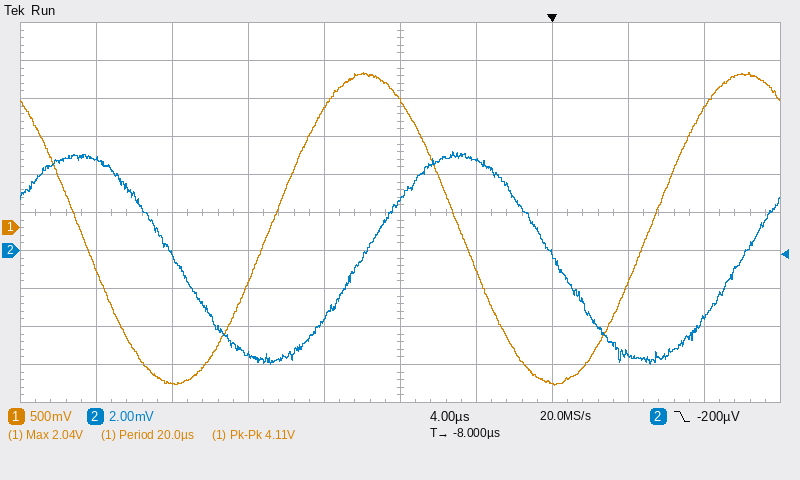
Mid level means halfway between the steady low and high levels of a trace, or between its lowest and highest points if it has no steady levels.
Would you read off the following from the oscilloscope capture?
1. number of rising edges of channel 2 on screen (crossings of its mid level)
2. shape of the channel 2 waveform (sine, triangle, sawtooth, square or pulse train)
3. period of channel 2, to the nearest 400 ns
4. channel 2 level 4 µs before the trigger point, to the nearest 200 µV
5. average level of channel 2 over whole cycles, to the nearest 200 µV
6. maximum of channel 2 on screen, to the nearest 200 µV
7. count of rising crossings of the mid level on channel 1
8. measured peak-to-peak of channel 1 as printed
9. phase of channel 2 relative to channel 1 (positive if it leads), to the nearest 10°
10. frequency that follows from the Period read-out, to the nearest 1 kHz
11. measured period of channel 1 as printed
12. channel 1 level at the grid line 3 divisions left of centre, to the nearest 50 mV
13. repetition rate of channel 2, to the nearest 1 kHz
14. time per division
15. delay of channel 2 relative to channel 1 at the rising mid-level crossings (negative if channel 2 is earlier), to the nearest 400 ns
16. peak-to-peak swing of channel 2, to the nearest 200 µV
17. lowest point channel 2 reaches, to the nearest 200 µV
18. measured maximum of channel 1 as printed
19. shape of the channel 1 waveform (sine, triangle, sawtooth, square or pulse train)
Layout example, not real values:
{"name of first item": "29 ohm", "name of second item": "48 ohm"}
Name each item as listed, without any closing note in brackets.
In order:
{"number of rising edges of channel 2 on screen": "2", "shape of the channel 2 waveform": "sine", "period of channel 2, to the nearest 400 ns": "20.0 µs", "channel 2 level 4 µs before the trigger point, to the nearest 200 µV": "4.8 mV", "average level of channel 2 over whole cycles, to the nearest 200 µV": "-400 µV", "maximum of channel 2 on screen, to the nearest 200 µV": "5.2 mV", "count of rising crossings of the mid level on channel 1": "2", "measured peak-to-peak of channel 1 as printed": "4.11 V", "phase of channel 2 relative to channel 1 (positive if it leads), to the nearest 10°": "-90°", "frequency that follows from the Period read-out, to the nearest 1 kHz": "50 kHz", "measured period of channel 1 as printed": "20.0 µs", "channel 1 level at the grid line 3 divisions left of centre, to the nearest 50 mV": "-2.05 V", "repetition rate of channel 2, to the nearest 1 kHz": "50 kHz", "time per division": "4 µs", "delay of channel 2 relative to channel 1 at the rising mid-level crossings (negative if channel 2 is earlier), to the nearest 400 ns": "+4.8 µs", "peak-to-peak swing of channel 2, to the nearest 200 µV": "11.2 mV", "lowest point channel 2 reaches, to the nearest 200 µV": "-6.0 mV", "measured maximum of channel 1 as printed": "2.04 V", "shape of the channel 1 waveform": "sine"}
